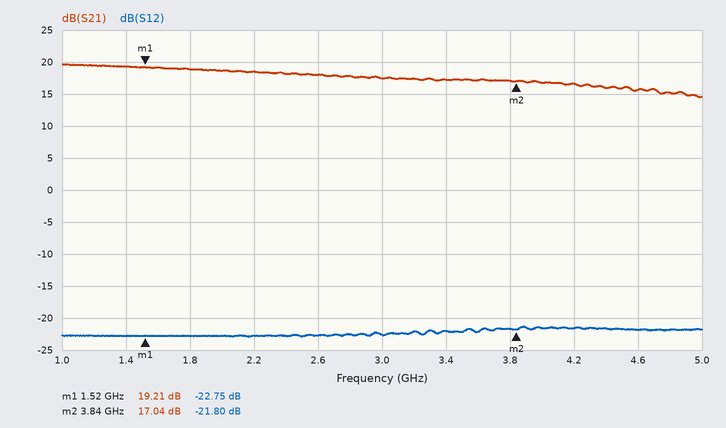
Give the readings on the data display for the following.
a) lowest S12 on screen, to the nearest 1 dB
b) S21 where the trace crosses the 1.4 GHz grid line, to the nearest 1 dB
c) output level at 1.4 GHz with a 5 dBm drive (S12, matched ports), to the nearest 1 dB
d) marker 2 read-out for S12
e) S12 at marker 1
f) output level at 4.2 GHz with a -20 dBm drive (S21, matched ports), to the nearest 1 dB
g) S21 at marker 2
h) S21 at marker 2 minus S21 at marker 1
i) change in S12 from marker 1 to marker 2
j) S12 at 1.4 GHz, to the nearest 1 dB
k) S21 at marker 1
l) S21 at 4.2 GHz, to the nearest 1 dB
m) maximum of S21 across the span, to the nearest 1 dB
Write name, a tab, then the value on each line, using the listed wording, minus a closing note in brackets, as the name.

lowest S12 on screen, to the nearest 1 dB	-23 dB
S21 where the trace crosses the 1.4 GHz grid line, to the nearest 1 dB	19 dB
output level at 1.4 GHz with a 5 dBm drive (S12, matched ports), to the nearest 1 dB	-18 dBm
marker 2 read-out for S12	-21.80 dB
S12 at marker 1	-22.75 dB
output level at 4.2 GHz with a -20 dBm drive (S21, matched ports), to the nearest 1 dB	-3 dBm
S21 at marker 2	17.04 dB
S21 at marker 2 minus S21 at marker 1	-2.17 dB
change in S12 from marker 1 to marker 2	0.95 dB
S12 at 1.4 GHz, to the nearest 1 dB	-23 dB
S21 at marker 1	19.21 dB
S21 at 4.2 GHz, to the nearest 1 dB	17 dB
maximum of S21 across the span, to the nearest 1 dB	20 dB
